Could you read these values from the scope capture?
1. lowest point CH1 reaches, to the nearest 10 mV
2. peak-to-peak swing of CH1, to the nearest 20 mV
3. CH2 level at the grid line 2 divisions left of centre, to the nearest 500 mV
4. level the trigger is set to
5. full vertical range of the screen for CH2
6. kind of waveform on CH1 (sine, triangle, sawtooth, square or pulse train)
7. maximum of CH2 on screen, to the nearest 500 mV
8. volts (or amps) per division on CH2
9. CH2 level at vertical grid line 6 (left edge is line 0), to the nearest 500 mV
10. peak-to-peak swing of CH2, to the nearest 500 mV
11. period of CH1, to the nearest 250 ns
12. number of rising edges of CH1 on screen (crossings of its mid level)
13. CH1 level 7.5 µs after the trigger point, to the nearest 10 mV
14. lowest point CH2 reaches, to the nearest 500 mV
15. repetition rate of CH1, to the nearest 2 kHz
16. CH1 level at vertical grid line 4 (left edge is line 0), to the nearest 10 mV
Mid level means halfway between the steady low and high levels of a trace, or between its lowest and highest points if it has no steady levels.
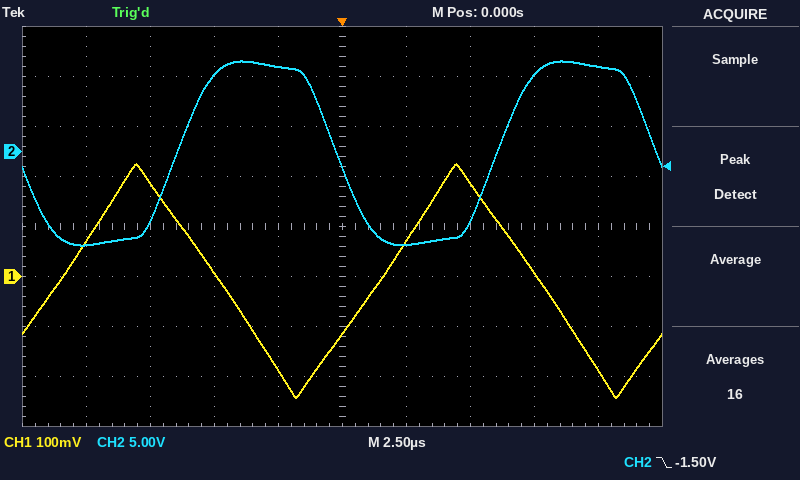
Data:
-240 mV
460 mV
7.5 V
-1.50 V
40 V
triangle
9.0 V
5 V
-9.5 V
18.5 V
12.50 µs
2
10 mV
-9.5 V
80 kHz
-190 mV
